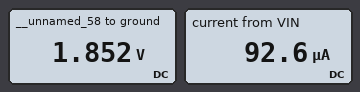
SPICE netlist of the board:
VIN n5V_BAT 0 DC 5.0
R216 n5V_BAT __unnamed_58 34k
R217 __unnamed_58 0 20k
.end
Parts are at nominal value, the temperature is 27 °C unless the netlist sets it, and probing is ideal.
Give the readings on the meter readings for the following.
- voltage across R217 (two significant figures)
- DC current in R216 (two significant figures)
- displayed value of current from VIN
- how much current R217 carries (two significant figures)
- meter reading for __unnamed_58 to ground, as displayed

1.9 V
93 µA
92.6 µA
93 µA
1.852 V
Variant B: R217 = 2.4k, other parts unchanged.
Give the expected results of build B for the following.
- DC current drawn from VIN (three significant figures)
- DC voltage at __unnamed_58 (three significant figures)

137 µA
330 mV
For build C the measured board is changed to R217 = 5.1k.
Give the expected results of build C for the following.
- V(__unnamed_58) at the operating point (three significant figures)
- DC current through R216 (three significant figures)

652 mV
128 µA
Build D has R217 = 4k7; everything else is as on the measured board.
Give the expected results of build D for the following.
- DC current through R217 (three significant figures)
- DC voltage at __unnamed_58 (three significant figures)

129 µA
607 mV
